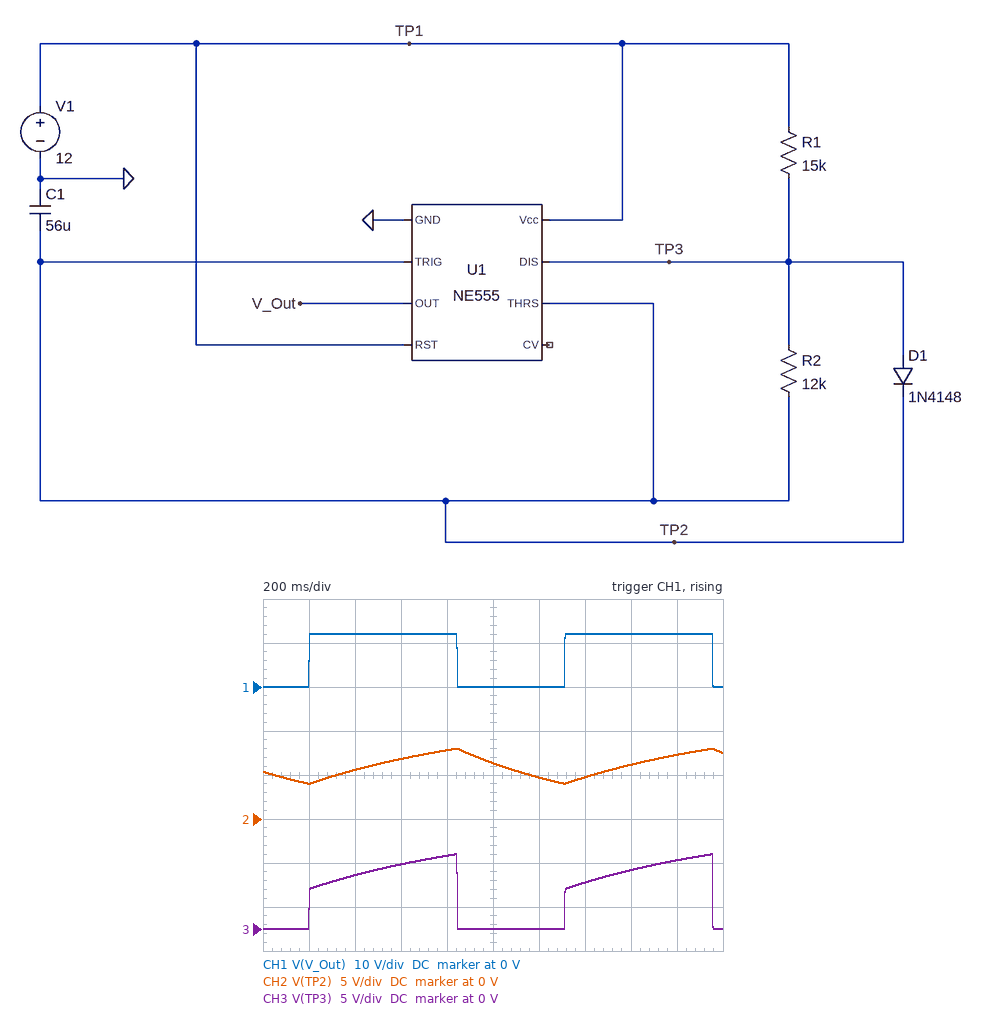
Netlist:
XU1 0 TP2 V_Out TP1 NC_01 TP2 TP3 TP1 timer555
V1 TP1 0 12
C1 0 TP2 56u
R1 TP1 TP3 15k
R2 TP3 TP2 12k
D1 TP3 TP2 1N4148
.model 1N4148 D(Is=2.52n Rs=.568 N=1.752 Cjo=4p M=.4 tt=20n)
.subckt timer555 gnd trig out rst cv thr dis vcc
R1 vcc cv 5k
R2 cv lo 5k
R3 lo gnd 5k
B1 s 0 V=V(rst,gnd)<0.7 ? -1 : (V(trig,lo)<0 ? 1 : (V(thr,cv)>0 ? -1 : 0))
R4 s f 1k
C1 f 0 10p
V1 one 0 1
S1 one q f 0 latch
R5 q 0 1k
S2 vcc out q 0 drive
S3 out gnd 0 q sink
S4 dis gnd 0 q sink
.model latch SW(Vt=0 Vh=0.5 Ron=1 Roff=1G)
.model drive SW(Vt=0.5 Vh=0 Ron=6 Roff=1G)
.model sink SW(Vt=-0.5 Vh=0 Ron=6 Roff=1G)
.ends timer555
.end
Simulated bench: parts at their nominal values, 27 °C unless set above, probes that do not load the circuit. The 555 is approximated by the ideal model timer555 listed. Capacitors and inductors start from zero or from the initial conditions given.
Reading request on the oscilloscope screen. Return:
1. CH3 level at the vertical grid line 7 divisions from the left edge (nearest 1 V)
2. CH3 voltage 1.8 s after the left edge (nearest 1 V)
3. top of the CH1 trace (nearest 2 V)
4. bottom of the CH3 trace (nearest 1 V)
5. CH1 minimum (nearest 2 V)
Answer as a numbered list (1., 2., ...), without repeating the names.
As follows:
1. 5 V
2. 8 V
3. 12 V
4. 0 V
5. 0 V
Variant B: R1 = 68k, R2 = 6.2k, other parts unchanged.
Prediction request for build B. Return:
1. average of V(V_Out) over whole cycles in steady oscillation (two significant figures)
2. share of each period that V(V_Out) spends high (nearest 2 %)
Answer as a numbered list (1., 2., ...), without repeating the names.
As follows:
1. 11 V
2. 92 %
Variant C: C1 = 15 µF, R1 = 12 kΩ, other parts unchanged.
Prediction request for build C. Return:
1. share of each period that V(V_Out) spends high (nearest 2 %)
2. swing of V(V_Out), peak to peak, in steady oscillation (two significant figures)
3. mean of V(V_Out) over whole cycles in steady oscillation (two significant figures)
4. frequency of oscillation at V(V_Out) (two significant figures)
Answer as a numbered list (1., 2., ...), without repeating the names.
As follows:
1. 52 %
2. 12 V
3. 6.3 V
4. 3.8 Hz
